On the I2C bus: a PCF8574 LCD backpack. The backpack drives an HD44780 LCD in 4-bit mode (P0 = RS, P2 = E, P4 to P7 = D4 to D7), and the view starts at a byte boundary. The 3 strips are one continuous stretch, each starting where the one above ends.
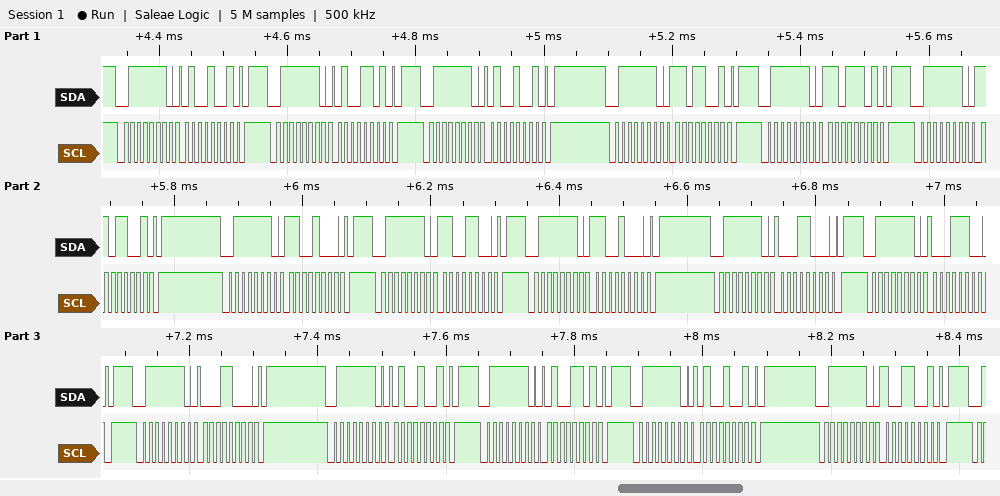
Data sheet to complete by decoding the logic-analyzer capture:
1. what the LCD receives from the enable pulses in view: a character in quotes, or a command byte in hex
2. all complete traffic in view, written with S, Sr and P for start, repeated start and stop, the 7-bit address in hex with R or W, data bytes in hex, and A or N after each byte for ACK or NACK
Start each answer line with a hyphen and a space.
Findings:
- 'M' 0xC1
- S 3FW A 49 A P S 3FW A 4D A P S 3FW A 49 A P S 3FW A D9 A P S 3FW A DD A P S 3FW A D9 A P S 3FW A C8 A P S 3FW A CC A P S 3FW A C8 A P S 3FW A 18 A P S 3FW A 1C A P S 3FW A 18 A P S 3FW A 49 A P S 3FW A 4D A P S 3FW A 49 A P S 3FW A 99 A P
